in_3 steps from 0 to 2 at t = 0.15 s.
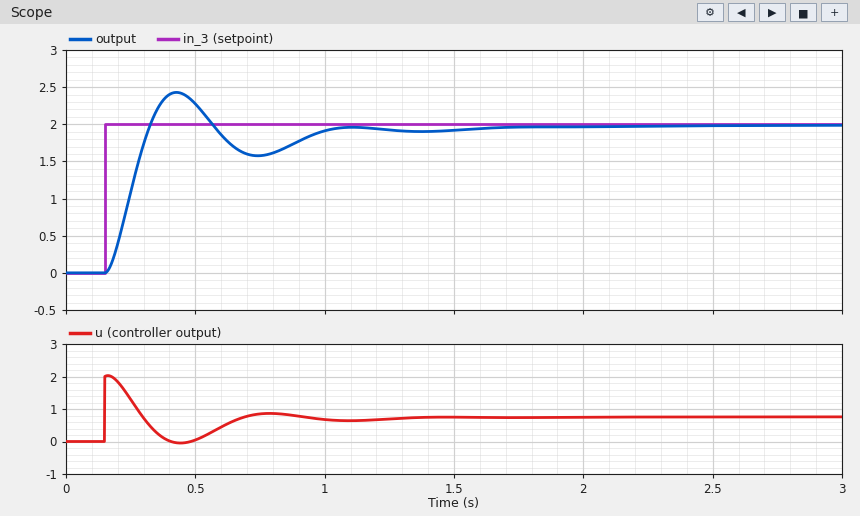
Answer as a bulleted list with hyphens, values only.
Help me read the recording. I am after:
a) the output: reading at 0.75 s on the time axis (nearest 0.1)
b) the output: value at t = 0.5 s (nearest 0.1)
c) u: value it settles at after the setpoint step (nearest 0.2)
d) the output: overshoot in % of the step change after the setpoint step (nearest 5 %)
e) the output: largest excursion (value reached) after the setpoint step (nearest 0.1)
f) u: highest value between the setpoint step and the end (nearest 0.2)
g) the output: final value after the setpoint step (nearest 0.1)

- 1.6
- 2.3
- 0.8
- 20 %
- 2.4
- 2.0
- 2.0
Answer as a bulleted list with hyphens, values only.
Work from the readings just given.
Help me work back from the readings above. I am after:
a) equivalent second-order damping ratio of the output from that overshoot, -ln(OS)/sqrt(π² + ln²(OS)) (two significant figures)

- 0.46
